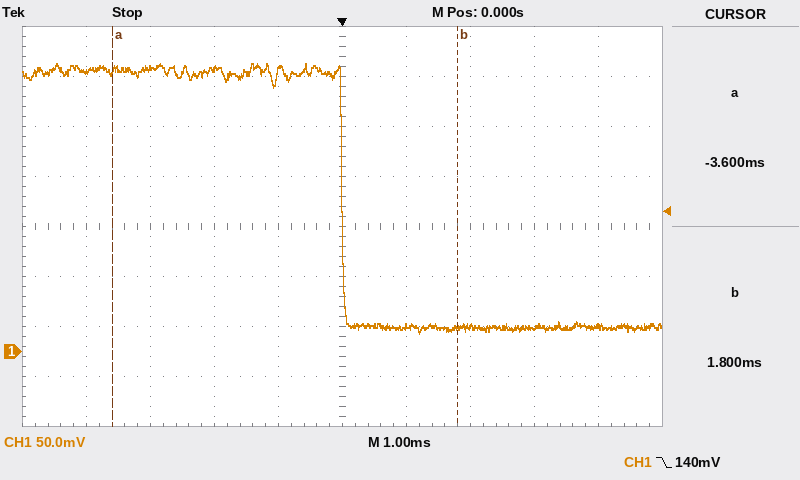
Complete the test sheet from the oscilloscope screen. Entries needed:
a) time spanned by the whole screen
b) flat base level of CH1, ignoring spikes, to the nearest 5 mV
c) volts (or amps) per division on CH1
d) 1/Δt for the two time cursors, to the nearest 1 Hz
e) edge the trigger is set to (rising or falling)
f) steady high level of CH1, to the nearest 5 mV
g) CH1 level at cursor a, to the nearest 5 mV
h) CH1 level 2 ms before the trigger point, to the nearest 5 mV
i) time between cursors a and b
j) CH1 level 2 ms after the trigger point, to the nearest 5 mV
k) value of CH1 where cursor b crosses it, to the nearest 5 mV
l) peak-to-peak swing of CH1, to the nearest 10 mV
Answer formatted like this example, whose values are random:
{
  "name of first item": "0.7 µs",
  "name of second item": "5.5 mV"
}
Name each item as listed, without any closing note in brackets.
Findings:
{
  "time spanned by the whole screen": "10 ms",
  "flat base level of CH1, ignoring spikes, to the nearest 5 mV": "25 mV",
  "volts (or amps) per division on CH1": "50 mV",
  "1/Δt for the two time cursors, to the nearest 1 Hz": "185 Hz",
  "edge the trigger is set to": "falling",
  "steady high level of CH1, to the nearest 5 mV": "280 mV",
  "CH1 level at cursor a, to the nearest 5 mV": "280 mV",
  "CH1 level 2 ms before the trigger point, to the nearest 5 mV": "285 mV",
  "time between cursors a and b": "5.4 ms",
  "CH1 level 2 ms after the trigger point, to the nearest 5 mV": "25 mV",
  "value of CH1 where cursor b crosses it, to the nearest 5 mV": "25 mV",
  "peak-to-peak swing of CH1, to the nearest 10 mV": "270 mV"
}
